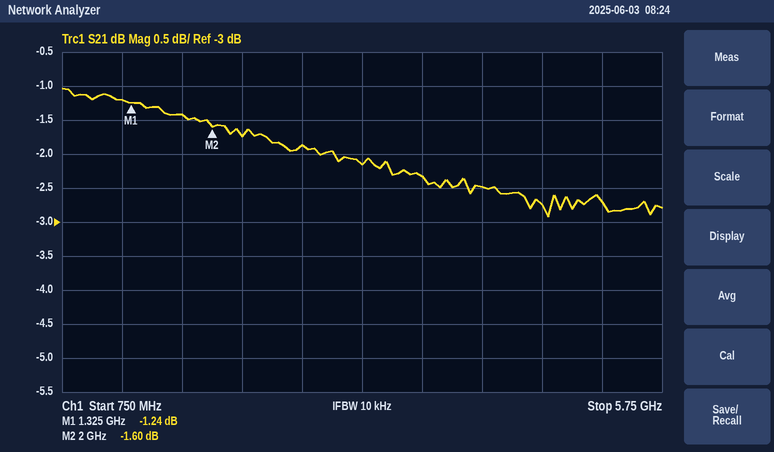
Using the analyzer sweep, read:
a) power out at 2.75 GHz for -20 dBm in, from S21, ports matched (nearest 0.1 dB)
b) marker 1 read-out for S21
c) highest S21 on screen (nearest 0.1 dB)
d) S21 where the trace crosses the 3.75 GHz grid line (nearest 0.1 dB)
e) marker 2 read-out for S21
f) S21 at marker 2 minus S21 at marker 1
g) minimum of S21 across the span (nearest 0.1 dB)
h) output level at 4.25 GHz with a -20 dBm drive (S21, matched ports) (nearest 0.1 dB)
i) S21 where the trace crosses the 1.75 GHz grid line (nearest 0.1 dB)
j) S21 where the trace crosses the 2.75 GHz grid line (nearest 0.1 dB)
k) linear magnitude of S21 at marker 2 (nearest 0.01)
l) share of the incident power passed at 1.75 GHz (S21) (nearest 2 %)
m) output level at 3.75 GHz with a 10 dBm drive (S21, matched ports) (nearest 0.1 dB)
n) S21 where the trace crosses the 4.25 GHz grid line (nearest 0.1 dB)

-21.9 dBm
-1.24 dB
-1.0 dB
-2.3 dB
-1.60 dB
-0.36 dB
-2.9 dB
-22.5 dBm
-1.4 dB
-1.9 dB
0.83
72 %
7.7 dBm
-2.5 dB
